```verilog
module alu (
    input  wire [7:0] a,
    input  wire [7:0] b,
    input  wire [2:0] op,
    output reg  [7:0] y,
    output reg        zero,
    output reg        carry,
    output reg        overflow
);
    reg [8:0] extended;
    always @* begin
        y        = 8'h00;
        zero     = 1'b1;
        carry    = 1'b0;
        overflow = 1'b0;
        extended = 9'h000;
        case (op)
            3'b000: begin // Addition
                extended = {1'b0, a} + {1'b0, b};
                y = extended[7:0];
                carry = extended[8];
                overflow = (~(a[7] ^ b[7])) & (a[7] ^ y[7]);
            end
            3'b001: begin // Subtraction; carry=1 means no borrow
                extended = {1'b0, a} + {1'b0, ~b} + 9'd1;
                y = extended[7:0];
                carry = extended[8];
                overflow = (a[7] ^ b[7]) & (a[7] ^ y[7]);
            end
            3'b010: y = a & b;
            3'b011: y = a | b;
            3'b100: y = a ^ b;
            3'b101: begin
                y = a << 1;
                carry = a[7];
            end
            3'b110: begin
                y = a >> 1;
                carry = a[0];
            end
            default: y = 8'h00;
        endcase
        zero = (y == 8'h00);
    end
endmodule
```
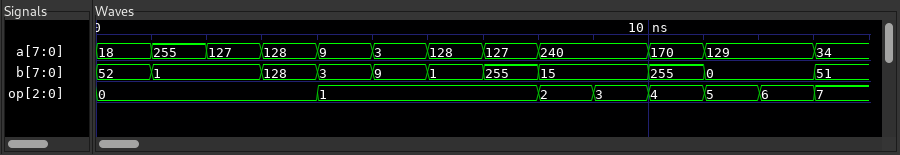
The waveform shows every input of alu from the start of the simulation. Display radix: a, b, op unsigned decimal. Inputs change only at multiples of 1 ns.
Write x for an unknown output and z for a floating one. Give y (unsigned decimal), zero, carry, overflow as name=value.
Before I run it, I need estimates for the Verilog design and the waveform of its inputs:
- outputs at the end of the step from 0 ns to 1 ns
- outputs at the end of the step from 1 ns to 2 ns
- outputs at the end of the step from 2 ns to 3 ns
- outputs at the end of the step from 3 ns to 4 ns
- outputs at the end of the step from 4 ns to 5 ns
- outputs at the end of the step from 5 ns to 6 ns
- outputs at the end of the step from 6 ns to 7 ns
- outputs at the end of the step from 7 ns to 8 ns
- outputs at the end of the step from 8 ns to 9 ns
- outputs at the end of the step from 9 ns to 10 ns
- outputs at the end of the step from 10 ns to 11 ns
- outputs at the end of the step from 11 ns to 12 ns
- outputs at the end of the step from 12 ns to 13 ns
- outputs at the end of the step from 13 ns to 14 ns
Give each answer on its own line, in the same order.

y=70, zero=0, carry=0, overflow=0
y=0, zero=1, carry=1, overflow=0
y=128, zero=0, carry=0, overflow=1
y=0, zero=1, carry=1, overflow=1
y=6, zero=0, carry=1, overflow=0
y=250, zero=0, carry=0, overflow=0
y=127, zero=0, carry=1, overflow=1
y=128, zero=0, carry=0, overflow=1
y=0, zero=1, carry=0, overflow=0
y=255, zero=0, carry=0, overflow=0
y=85, zero=0, carry=0, overflow=0
y=2, zero=0, carry=1, overflow=0
y=64, zero=0, carry=1, overflow=0
y=0, zero=1, carry=0, overflow=0
